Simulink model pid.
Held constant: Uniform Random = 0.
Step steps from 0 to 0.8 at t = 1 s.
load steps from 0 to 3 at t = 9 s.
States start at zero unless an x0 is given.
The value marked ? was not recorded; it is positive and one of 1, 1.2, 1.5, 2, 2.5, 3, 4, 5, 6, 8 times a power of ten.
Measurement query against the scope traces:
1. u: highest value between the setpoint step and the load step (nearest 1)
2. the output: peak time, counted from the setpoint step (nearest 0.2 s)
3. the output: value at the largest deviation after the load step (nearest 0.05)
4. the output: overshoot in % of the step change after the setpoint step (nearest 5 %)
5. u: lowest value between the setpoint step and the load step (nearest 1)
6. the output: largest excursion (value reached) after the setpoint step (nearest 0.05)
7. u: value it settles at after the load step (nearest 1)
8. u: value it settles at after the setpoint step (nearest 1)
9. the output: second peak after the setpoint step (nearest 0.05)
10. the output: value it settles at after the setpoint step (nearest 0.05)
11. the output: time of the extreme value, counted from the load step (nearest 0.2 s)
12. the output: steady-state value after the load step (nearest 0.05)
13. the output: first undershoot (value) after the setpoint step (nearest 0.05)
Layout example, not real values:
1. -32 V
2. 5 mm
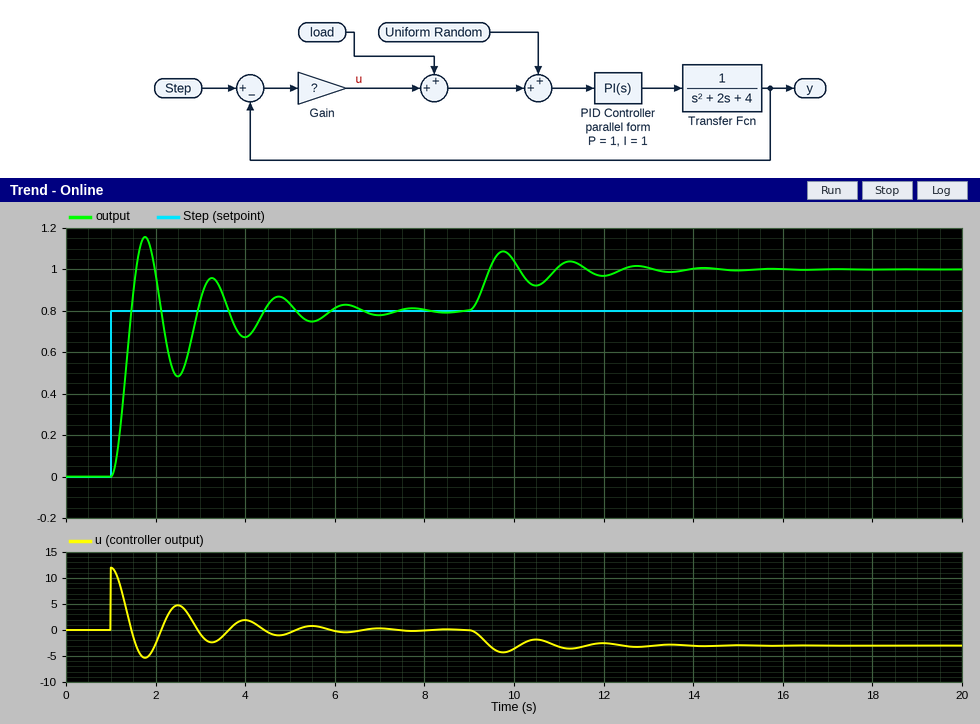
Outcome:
1. 12
2. 0.8 s
3. 1.10
4. 45 %
5. -5
6. 1.15
7. -3
8. 0
9. 0.95
10. 0.80
11. 0.8 s
12. 1.00
13. 0.50
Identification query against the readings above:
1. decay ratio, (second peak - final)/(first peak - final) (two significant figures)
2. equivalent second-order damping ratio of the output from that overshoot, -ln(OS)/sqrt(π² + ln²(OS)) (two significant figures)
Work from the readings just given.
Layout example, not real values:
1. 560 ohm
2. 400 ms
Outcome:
1. 0.43
2. 0.25
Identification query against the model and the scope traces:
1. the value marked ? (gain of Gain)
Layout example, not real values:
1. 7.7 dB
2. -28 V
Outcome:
1. 15
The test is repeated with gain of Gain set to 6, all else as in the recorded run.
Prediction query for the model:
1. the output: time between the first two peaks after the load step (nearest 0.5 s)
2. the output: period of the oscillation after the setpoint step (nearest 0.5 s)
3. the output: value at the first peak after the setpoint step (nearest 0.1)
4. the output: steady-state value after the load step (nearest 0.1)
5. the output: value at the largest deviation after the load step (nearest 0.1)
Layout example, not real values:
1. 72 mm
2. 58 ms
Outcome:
1. 2.0 s
2. 2.0 s
3. 0.9
4. 1.3
5. 1.4
